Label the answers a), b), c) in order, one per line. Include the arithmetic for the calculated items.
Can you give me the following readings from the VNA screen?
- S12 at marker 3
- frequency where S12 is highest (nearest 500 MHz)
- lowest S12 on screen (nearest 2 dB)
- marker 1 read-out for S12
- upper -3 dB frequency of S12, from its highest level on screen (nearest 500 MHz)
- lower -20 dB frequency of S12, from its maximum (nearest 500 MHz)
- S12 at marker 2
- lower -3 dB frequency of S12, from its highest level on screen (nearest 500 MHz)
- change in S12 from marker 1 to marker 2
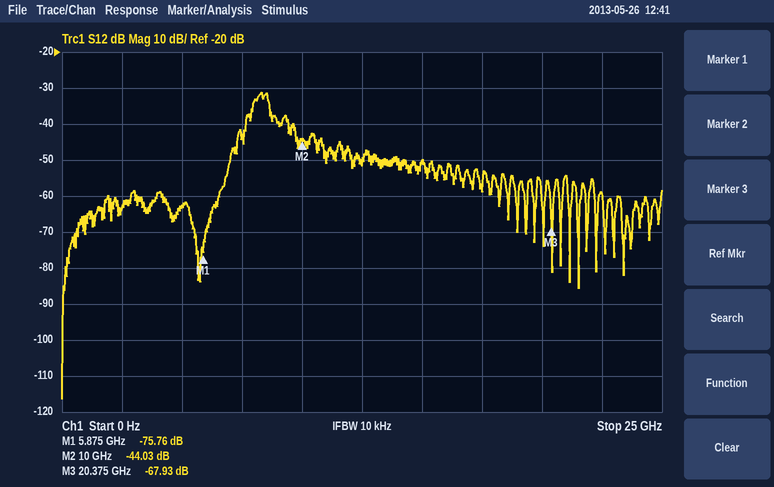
a) -67.93 dB
b) 8.5 GHz
c) -116 dB
d) -75.76 dB
e) 8.5 GHz
f) 7.0 GHz
g) -44.03 dB
h) 8.0 GHz
i) -44.03 − (-75.76) = 31.73 dB
